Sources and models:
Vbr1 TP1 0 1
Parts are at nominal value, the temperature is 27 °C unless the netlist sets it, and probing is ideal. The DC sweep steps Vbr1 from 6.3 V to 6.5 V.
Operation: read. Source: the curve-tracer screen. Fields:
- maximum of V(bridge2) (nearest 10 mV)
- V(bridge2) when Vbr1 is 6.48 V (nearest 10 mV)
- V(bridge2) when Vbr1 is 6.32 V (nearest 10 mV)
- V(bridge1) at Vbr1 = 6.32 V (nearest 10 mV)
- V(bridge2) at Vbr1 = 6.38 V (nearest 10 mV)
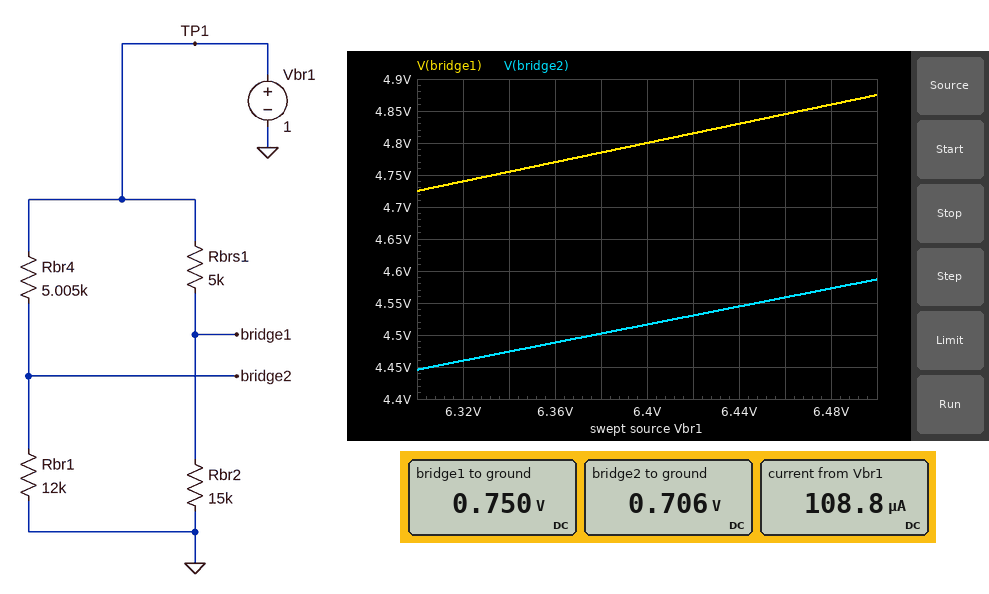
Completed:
4.59 V
4.57 V
4.46 V
4.74 V
4.50 V
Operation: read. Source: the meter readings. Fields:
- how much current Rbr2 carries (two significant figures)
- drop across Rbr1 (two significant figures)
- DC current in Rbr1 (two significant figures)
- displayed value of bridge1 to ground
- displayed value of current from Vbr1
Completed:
50 µA
710 mV
59 µA
0.750 V
108.8 µA
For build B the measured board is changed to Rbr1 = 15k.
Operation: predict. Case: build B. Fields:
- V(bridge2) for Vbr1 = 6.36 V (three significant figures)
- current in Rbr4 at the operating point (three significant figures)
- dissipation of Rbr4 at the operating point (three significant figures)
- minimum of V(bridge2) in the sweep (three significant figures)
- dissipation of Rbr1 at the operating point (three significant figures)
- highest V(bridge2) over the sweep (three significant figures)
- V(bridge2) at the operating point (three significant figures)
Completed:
4.77 V
50.0 µA
12.5 µW
4.72 V
37.5 µW
4.87 V
750 mV
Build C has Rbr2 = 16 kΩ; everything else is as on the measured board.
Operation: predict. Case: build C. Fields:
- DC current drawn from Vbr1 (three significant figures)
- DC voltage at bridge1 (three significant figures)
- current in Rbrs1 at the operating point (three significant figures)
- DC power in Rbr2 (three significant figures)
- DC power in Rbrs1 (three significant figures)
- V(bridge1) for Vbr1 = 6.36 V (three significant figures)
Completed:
106 µA
762 mV
47.6 µA
36.3 µW
11.3 µW
4.85 V
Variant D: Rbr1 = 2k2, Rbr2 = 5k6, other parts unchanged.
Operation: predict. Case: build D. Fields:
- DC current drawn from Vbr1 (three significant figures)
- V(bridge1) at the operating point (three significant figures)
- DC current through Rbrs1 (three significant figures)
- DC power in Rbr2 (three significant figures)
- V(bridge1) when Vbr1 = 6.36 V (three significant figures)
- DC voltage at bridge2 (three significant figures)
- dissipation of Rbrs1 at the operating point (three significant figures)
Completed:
233 µA
528 mV
94.3 µA
49.8 µW
3.36 V
305 mV
44.5 µW
